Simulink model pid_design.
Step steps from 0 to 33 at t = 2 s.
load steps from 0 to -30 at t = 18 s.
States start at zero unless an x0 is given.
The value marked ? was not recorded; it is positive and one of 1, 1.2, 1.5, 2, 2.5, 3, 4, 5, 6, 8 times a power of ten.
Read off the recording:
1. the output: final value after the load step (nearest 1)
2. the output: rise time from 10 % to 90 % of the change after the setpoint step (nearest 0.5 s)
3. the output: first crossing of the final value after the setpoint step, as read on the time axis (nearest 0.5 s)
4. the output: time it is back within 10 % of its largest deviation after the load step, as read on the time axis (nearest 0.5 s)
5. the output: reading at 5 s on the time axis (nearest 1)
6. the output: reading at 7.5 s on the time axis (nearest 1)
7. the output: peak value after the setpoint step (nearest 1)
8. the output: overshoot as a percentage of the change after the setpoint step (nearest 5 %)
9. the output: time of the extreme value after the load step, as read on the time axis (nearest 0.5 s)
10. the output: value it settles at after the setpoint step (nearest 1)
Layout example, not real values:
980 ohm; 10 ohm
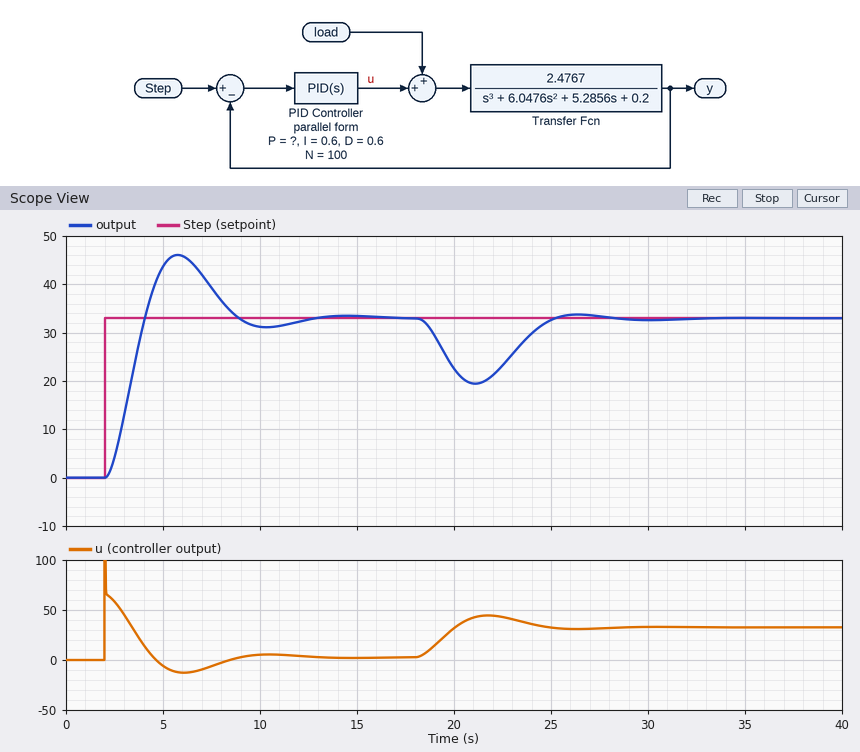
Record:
33; 1.5 s; 4.0 s; 24.5 s; 44; 39; 46; 40 %; 21.0 s; 33
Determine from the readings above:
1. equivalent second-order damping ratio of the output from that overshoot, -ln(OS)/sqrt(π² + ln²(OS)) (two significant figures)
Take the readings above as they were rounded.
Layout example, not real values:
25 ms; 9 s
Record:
0.28
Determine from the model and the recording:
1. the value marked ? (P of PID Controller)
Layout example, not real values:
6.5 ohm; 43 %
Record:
2
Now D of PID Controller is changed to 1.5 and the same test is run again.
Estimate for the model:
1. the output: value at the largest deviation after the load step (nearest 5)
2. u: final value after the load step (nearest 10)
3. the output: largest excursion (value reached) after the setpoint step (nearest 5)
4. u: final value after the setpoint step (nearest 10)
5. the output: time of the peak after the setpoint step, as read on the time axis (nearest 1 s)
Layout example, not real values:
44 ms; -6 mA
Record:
20; 30; 40; 0; 6 s
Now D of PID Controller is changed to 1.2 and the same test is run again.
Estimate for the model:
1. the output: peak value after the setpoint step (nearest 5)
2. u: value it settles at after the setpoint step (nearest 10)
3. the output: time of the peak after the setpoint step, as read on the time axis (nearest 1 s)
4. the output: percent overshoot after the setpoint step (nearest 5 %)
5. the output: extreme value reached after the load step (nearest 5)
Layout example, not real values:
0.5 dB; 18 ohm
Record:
40; 0; 6 s; 25 %; 20
